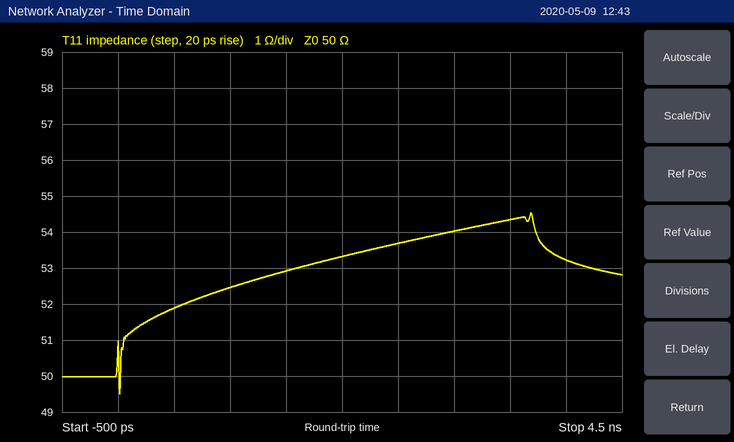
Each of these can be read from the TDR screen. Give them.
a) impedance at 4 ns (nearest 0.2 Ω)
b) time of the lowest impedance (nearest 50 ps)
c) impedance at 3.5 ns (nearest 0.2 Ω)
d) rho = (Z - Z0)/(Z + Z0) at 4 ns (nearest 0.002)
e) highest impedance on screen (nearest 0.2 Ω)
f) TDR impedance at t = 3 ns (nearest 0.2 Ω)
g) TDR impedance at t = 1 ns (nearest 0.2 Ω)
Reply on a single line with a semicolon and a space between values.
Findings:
53.2 Ω; 0 ps; 54.4 Ω; +0.032; 54.6 Ω; 54.0 Ω; 52.4 Ω
